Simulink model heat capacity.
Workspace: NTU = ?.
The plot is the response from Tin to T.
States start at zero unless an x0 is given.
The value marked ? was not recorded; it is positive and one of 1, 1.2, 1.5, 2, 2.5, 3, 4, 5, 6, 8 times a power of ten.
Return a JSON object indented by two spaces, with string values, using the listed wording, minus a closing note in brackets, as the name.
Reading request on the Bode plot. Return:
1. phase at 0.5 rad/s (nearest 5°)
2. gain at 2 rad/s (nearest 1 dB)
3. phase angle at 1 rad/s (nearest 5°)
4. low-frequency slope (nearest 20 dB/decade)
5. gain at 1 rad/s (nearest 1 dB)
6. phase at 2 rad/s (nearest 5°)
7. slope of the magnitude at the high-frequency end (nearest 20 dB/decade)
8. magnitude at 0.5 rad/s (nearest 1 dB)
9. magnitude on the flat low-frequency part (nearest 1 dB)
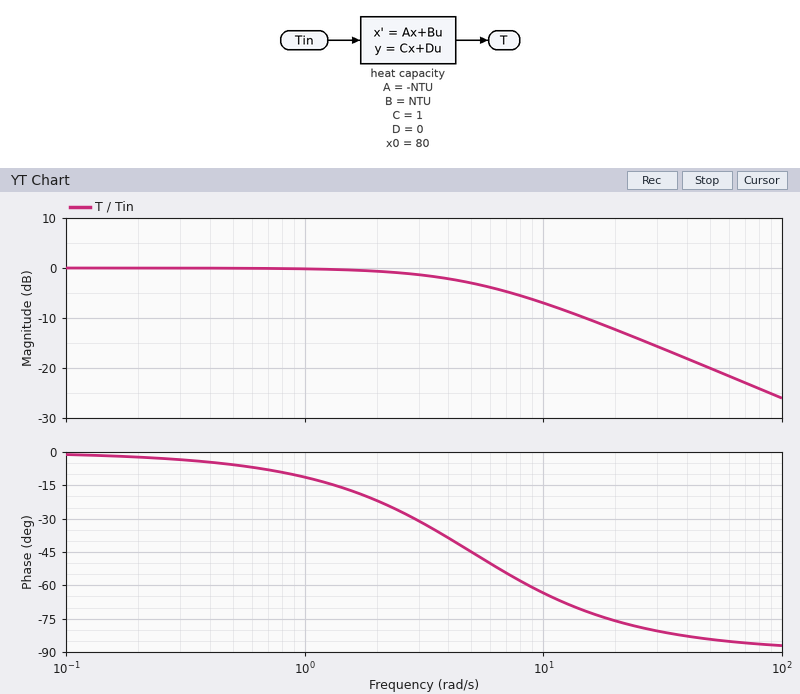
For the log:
{
  "phase at 0.5 rad/s": "-5°",
  "gain at 2 rad/s": "-1 dB",
  "phase angle at 1 rad/s": "-10°",
  "low-frequency slope": "0 dB/decade",
  "gain at 1 rad/s": "0 dB",
  "phase at 2 rad/s": "-20°",
  "slope of the magnitude at the high-frequency end": "-20 dB/decade",
  "magnitude at 0.5 rad/s": "0 dB",
  "magnitude on the flat low-frequency part": "0 dB"
}
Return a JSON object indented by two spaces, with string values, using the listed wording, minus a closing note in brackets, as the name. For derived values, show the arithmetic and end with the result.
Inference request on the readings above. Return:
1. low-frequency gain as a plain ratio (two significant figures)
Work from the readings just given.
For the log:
{
  "low-frequency gain as a plain ratio": "10^(0 / 20) = 1.0"
}
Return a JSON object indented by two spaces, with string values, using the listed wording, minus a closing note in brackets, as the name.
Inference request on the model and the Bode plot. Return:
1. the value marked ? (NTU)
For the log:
{
  "the value marked ?": "5"
}
